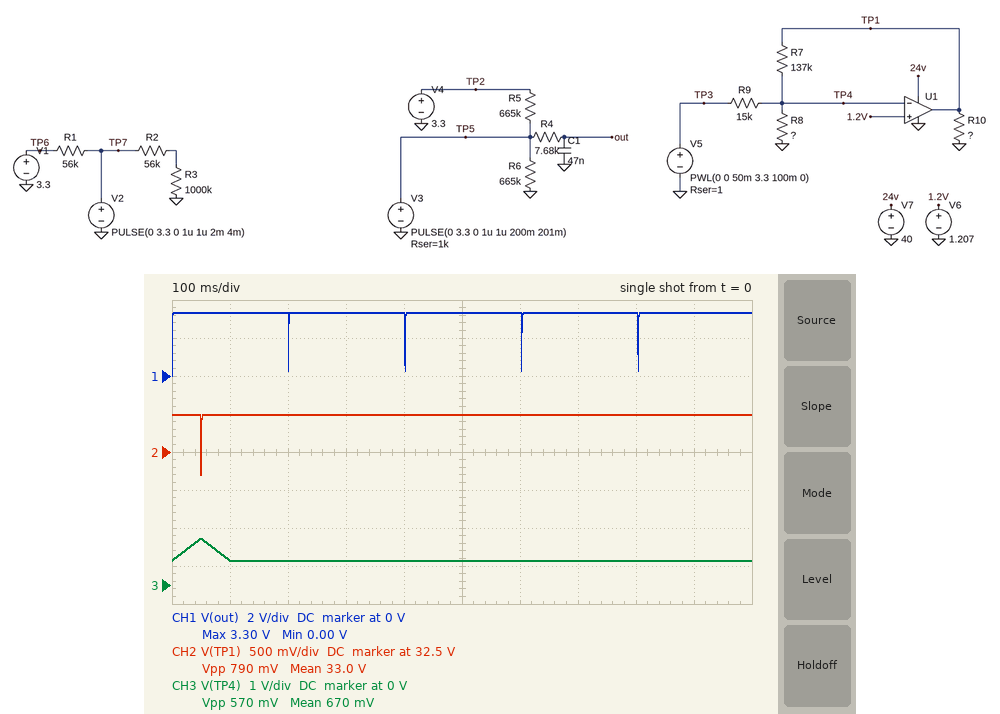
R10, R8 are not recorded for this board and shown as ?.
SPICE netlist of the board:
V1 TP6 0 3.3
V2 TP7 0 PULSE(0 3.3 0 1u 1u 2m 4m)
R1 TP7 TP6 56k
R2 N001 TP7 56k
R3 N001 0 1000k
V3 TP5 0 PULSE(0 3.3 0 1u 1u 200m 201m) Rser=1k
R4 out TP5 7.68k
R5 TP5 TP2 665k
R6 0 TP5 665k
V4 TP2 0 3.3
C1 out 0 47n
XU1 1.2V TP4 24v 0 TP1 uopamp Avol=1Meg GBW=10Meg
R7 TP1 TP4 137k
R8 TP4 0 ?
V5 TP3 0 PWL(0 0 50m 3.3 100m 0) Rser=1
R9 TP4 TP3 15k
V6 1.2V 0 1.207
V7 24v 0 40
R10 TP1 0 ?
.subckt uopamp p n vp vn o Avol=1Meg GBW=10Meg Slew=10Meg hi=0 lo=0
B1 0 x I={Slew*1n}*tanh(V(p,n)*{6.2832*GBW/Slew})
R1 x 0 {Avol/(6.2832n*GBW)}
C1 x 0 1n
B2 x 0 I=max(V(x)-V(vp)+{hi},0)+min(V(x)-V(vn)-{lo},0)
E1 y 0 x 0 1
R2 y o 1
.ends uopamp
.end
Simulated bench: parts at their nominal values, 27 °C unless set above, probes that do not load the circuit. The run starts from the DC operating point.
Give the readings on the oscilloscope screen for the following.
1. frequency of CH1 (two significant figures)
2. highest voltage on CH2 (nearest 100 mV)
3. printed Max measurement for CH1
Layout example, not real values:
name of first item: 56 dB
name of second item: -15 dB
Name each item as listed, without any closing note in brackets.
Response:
frequency of CH1: 5.0 Hz
highest voltage on CH2: 33.0 V
printed Max measurement for CH1: 3.30 V
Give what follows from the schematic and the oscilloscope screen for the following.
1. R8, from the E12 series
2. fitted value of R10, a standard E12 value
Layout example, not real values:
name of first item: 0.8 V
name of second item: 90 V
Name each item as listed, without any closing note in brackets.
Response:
R8, from the E12 series: 3.3 kΩ
fitted value of R10, a standard E12 value: 4.7 Ω
